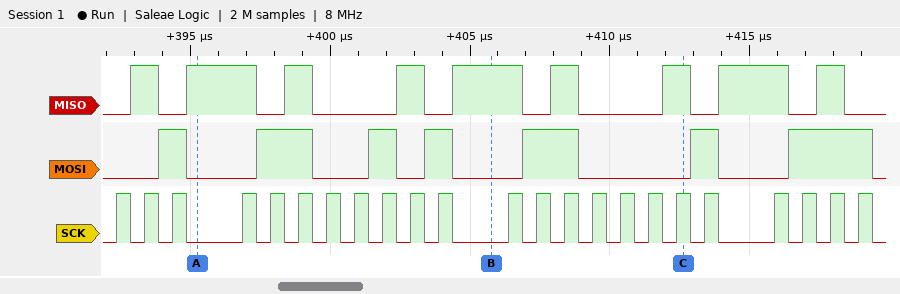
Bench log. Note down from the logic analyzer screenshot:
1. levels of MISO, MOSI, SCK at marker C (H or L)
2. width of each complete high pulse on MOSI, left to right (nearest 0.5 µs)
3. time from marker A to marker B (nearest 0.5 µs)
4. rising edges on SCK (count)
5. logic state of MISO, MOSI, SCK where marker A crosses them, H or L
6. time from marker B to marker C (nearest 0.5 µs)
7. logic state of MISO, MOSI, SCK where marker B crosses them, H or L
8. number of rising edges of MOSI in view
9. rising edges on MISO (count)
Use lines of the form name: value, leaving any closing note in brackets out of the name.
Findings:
levels of MISO, MOSI, SCK at marker C: MISO=H, MOSI=L, SCK=H
width of each complete high pulse on MOSI, left to right: 1 µs, 2 µs, 1 µs, 1 µs, 2 µs, 1 µs, 3 µs
time from marker A to marker B: 10.5 µs
rising edges on SCK: 23
logic state of MISO, MOSI, SCK where marker A crosses them, H or L: MISO=H, MOSI=L, SCK=L
time from marker B to marker C: 7 µs
logic state of MISO, MOSI, SCK where marker B crosses them, H or L: MISO=H, MOSI=L, SCK=L
number of rising edges of MOSI in view: 7
rising edges on MISO: 9
